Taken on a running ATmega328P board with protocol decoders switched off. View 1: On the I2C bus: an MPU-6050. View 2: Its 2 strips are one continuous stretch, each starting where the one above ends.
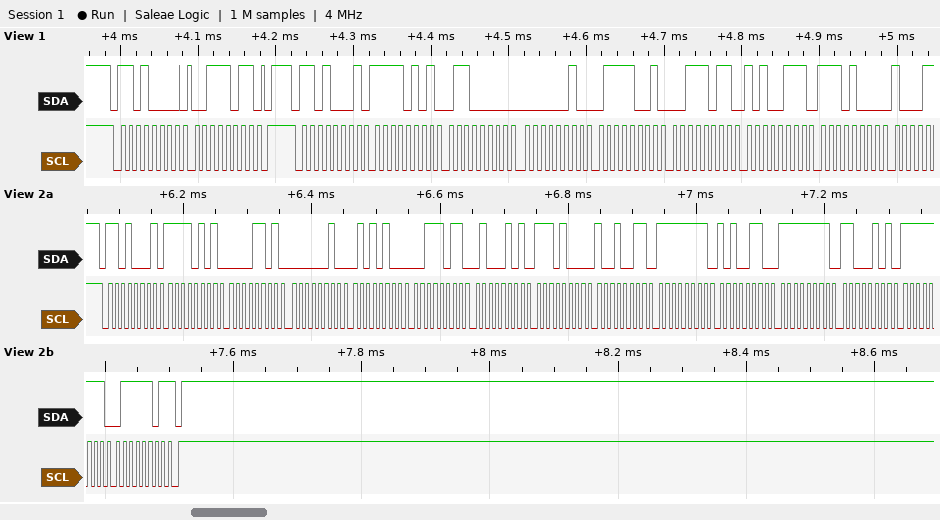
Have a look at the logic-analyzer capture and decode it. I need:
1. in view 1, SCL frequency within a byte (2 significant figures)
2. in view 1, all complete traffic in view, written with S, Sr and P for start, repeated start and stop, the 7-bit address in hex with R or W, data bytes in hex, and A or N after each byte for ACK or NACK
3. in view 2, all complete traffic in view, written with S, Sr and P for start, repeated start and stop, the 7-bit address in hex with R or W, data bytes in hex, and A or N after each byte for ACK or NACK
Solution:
100 kHz
S 68W A 3B A P S 68R A F5 A 60 A 02 A 79 A 3B A A7 A E8 A
S 68R A F5 A 0D A 02 A 54 A 3B A 45 A E8 A 93 A FF A A6 A FF A C5 A FF A 7D N P
